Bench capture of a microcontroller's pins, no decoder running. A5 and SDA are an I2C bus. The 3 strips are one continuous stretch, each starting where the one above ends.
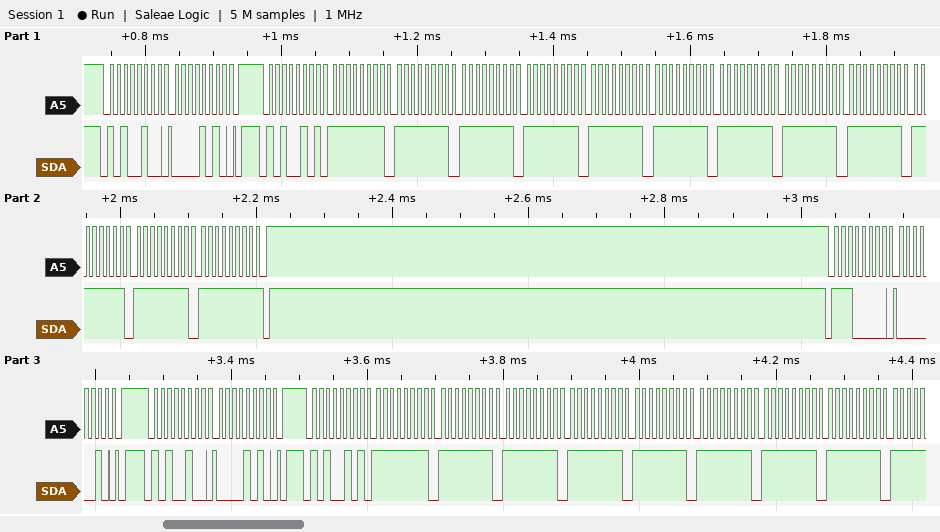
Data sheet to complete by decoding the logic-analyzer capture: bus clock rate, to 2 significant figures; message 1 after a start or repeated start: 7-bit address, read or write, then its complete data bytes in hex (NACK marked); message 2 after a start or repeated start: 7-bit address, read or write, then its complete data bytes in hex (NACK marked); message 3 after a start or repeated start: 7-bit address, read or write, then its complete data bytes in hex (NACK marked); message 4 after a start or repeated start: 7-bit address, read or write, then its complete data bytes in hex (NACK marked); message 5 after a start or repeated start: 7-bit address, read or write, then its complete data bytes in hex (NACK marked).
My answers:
100 kHz
0x52 write: 0A
0x52 read: FF FF FF FF FF FF FF FF FF FF FF FF NACK
0x70 write: 02
0x52 write: 0A
0x52 read: FF FF FF FF FF FF FF FF
